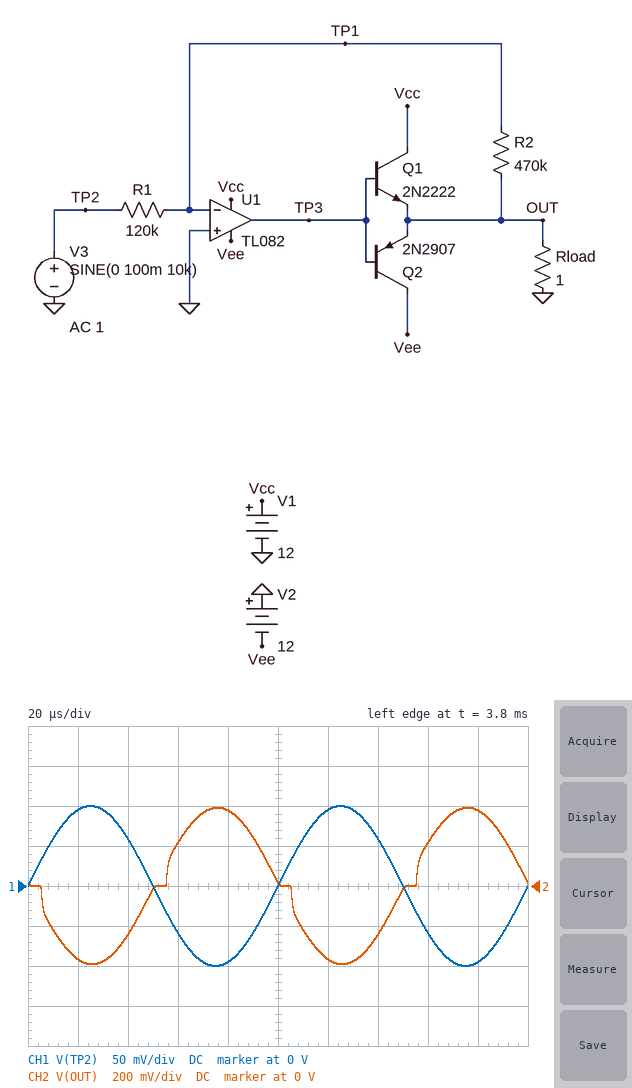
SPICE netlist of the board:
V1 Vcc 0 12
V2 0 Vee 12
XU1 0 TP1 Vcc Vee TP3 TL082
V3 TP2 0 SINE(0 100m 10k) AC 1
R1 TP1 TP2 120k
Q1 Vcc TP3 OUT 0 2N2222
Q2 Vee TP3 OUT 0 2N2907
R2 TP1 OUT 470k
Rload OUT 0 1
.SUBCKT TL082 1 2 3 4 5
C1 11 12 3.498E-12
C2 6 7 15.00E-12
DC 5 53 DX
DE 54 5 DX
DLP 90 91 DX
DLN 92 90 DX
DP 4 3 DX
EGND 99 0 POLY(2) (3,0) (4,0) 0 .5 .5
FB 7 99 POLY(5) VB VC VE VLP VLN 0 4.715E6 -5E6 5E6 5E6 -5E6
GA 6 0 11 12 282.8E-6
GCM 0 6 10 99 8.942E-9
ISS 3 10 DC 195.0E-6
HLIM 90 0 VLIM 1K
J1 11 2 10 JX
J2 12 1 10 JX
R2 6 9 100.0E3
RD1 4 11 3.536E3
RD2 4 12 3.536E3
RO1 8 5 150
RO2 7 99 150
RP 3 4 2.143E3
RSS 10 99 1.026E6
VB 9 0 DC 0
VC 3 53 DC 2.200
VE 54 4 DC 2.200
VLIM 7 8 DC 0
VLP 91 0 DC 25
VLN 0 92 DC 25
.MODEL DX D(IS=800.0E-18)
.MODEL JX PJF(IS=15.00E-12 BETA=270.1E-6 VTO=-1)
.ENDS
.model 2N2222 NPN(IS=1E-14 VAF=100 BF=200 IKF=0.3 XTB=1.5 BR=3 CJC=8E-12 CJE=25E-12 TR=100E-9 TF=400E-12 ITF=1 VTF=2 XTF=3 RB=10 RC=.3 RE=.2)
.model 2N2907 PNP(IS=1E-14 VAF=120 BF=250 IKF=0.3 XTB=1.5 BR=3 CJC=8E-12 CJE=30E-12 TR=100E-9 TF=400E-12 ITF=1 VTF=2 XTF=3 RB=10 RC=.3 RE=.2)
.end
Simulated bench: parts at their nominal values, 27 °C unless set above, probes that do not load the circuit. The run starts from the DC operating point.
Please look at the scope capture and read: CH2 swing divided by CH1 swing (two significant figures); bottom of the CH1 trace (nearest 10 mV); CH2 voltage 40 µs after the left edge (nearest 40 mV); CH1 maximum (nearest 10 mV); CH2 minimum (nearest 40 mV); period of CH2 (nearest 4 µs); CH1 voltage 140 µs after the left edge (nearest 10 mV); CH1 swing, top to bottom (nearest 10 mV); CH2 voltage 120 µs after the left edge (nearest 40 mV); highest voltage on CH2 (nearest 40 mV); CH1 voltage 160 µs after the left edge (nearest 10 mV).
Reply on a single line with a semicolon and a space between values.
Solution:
3.9; -100 mV; -240 mV; 100 mV; -400 mV; 100 µs; 60 mV; 200 mV; -360 mV; 400 mV; -60 mV
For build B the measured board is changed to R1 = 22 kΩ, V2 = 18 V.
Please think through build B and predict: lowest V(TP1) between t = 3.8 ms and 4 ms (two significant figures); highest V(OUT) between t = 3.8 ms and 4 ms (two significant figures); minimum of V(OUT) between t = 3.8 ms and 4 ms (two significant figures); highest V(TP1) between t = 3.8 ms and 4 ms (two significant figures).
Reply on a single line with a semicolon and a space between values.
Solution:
-41 mV; 1.2 V; -1.4 V; 35 mV
